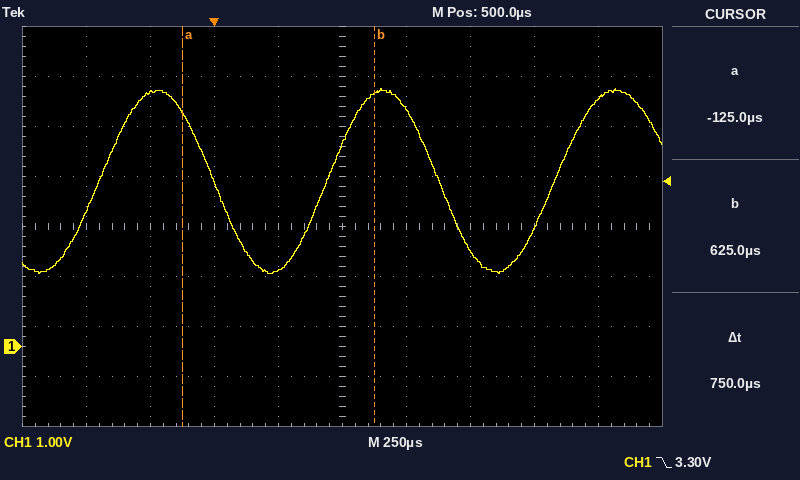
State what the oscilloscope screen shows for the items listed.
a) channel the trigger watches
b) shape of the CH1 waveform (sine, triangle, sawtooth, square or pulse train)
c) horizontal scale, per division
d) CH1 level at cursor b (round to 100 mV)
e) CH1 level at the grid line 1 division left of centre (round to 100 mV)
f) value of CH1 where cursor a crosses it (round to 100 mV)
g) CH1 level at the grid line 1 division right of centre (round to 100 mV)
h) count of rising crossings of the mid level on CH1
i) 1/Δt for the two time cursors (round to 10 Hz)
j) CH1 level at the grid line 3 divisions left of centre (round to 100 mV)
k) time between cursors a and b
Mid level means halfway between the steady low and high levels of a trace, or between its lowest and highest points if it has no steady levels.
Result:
CH1
sine
250 µs
5.1 V
1.5 V
4.7 V
4.7 V
3
1.33 kHz
5.1 V
750 µs
